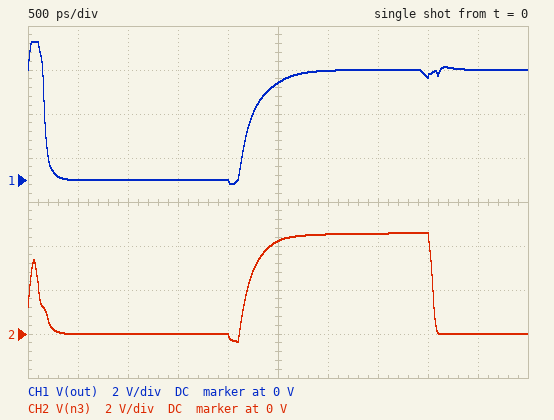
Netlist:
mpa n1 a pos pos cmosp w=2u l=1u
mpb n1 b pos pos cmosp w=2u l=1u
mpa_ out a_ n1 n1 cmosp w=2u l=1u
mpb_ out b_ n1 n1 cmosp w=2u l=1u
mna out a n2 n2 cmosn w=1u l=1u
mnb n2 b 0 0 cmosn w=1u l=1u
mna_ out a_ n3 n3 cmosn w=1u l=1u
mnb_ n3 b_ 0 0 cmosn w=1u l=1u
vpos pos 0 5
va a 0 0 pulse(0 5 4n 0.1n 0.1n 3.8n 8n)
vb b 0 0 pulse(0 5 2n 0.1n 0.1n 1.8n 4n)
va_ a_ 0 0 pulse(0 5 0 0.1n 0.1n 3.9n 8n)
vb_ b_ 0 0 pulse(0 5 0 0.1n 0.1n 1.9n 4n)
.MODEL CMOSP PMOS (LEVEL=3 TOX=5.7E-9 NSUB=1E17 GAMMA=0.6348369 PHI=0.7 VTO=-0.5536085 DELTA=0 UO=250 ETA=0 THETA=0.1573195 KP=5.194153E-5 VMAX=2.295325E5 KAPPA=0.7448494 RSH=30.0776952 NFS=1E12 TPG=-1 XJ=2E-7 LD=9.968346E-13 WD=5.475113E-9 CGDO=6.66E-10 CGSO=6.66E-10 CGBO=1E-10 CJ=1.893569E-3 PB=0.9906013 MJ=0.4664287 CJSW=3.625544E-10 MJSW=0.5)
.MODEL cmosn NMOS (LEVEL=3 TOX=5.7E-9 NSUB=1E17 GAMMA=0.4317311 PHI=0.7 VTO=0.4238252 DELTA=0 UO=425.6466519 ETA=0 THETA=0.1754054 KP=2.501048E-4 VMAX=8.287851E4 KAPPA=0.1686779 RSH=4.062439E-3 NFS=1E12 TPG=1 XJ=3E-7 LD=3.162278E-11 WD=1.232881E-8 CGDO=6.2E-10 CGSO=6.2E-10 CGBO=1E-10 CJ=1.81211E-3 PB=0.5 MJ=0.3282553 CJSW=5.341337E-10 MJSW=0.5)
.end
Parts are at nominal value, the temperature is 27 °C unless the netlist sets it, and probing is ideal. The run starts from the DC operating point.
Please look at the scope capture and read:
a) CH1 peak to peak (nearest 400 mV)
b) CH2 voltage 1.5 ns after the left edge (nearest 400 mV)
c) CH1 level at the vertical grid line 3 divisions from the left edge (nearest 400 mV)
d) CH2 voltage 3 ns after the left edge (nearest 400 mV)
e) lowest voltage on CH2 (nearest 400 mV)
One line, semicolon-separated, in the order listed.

6.4 V; 0 V; 0 V; 4.4 V; -400 mV
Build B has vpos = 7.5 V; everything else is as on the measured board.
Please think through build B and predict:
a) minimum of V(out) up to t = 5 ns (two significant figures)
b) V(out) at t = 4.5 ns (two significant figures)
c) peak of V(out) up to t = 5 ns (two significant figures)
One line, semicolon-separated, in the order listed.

600 mV; 7.5 V; 8.8 V
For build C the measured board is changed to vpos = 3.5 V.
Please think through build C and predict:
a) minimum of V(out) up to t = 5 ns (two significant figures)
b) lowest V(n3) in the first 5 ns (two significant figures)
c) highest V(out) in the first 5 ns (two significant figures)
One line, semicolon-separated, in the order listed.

-380 mV; -590 mV; 4.8 V
